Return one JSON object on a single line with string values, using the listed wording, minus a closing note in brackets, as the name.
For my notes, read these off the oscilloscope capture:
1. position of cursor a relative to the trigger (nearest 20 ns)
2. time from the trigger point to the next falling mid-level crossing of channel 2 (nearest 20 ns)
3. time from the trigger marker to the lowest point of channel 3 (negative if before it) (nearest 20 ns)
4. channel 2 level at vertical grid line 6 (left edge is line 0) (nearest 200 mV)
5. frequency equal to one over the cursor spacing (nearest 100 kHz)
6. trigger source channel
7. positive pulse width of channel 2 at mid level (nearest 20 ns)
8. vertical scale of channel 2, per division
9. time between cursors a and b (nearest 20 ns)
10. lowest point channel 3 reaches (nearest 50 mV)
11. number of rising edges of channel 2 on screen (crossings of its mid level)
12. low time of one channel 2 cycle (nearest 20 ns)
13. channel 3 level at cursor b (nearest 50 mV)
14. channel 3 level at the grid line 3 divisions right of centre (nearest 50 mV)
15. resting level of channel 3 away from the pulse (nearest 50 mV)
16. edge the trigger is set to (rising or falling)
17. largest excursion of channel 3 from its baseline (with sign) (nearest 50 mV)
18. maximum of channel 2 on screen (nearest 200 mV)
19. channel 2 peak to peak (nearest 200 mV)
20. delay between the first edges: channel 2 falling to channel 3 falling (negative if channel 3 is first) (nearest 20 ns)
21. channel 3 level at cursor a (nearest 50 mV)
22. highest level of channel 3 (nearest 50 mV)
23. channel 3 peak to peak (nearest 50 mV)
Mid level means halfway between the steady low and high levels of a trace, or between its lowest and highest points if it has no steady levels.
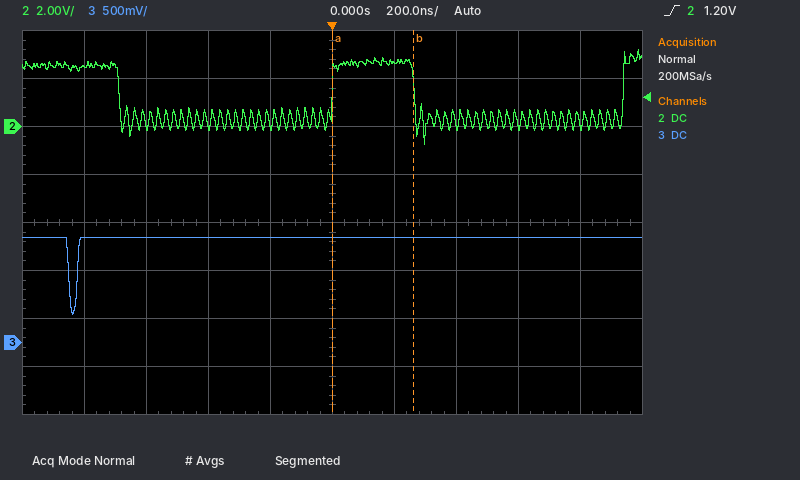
{"position of cursor a relative to the trigger": "0 ns", "time from the trigger point to the next falling mid-level crossing of channel 2": "260 ns", "time from the trigger marker to the lowest point of channel 3 (negative if before it)": "-840 ns", "channel 2 level at vertical grid line 6 (left edge is line 0)": "2.6 V", "frequency equal to one over the cursor spacing": "3.8 MHz", "trigger source channel": "channel 2", "positive pulse width of channel 2 at mid level": "260 ns", "vertical scale of channel 2, per division": "2 V", "time between cursors a and b": "260 ns", "lowest point channel 3 reaches": "300 mV", "number of rising edges of channel 2 on screen": "2", "low time of one channel 2 cycle": "680 ns", "channel 3 level at cursor b": "1.10 V", "channel 3 level at the grid line 3 divisions right of centre": "1.10 V", "resting level of channel 3 away from the pulse": "1.10 V", "edge the trigger is set to": "rising", "largest excursion of channel 3 from its baseline (with sign)": "-800 mV", "maximum of channel 2 on screen": "3.2 V", "channel 2 peak to peak": "4.0 V", "delay between the first edges: channel 2 falling to channel 3 falling (negative if channel 3 is first)": "-160 ns", "channel 3 level at cursor a": "1.10 V", "highest level of channel 3": "1.10 V", "channel 3 peak to peak": "800 mV"}
